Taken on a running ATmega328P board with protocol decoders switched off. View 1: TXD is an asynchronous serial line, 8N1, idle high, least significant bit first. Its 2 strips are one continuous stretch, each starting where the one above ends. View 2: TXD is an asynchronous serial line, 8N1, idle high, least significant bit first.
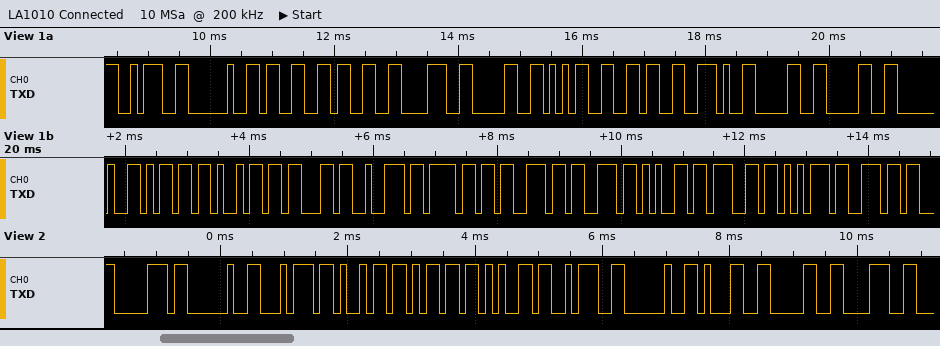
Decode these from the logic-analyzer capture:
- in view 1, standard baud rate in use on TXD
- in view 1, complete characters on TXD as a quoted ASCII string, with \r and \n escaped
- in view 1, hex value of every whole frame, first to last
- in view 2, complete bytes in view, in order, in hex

9600 baud
": 338056.00 microssegun"
3A 20 33 33 38 30 35 36 2E 30 30 20 6D 69 63 72 6F 73 73 65 67 75 6E
70 20 74 69 6D 65 3A 20 31 30 38
